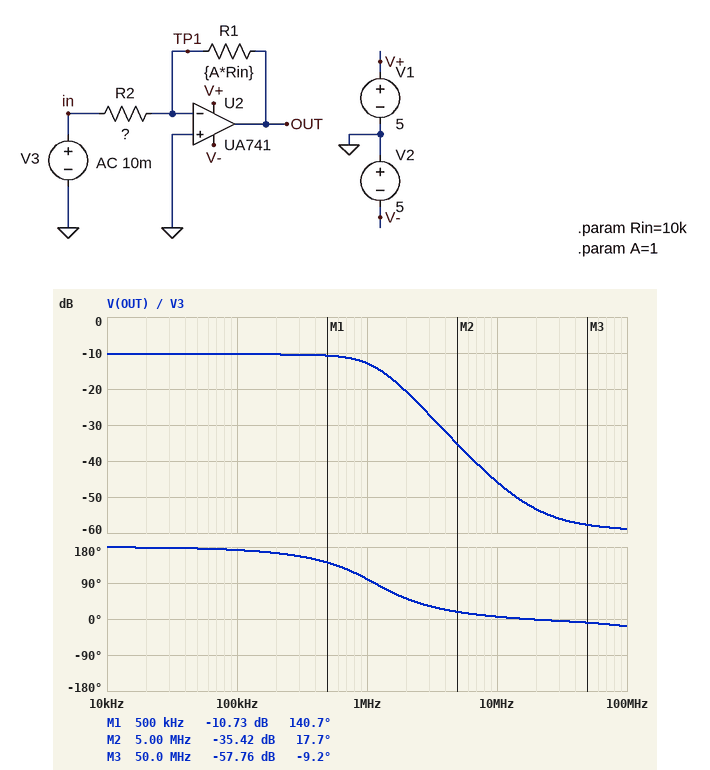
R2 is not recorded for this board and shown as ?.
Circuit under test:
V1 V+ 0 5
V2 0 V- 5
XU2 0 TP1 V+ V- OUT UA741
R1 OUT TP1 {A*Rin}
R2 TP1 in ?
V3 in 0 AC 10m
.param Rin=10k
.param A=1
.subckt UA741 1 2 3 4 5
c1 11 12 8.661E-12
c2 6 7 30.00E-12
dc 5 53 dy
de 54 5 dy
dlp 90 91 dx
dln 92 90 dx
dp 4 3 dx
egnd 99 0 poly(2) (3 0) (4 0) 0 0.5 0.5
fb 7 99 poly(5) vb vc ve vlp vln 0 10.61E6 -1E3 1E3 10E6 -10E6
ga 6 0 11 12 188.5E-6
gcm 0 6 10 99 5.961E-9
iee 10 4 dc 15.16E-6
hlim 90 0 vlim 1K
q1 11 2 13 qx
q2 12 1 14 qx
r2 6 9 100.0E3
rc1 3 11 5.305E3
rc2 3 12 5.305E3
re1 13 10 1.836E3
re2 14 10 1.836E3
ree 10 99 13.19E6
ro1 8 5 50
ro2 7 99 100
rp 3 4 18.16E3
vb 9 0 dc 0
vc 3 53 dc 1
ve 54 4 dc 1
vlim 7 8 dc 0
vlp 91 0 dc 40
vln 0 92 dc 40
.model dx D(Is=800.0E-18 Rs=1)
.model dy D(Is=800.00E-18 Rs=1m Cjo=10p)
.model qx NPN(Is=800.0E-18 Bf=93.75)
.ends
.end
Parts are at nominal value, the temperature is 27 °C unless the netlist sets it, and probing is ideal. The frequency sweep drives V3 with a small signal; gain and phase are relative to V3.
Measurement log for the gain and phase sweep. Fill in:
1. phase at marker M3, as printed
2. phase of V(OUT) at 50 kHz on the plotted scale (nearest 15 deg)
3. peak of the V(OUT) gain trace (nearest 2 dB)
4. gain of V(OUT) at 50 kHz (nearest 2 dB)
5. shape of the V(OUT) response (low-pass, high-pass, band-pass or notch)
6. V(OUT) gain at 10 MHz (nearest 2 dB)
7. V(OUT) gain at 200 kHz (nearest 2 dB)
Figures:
-9.2 deg
180 deg
-10 dB
-10 dB
low-pass
-46 dB
-10 dB
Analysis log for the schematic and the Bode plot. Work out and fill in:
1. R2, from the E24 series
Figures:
33 kΩ
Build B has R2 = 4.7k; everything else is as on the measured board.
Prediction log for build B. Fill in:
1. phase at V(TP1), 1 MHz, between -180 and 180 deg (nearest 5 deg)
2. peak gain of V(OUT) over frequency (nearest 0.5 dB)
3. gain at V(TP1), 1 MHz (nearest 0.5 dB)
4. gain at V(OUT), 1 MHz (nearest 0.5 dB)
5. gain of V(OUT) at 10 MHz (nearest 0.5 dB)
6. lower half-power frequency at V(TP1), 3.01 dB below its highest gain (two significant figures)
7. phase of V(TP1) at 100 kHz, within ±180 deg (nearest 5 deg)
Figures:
15 deg
6.5 dB
-2.5 dB
-3.5 dB
-36.5 dB
320 kHz
75 deg
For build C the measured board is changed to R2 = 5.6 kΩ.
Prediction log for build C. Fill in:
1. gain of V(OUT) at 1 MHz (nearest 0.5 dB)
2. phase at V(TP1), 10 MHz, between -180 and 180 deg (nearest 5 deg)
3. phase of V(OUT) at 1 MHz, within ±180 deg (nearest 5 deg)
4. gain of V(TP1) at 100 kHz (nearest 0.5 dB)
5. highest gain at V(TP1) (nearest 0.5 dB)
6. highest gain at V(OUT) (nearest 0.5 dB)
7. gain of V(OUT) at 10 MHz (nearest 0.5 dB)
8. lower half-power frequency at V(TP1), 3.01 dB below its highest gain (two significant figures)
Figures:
-4.0 dB
0 deg
75 deg
-15.0 dB
-3.0 dB
5.0 dB
-37.0 dB
360 kHz
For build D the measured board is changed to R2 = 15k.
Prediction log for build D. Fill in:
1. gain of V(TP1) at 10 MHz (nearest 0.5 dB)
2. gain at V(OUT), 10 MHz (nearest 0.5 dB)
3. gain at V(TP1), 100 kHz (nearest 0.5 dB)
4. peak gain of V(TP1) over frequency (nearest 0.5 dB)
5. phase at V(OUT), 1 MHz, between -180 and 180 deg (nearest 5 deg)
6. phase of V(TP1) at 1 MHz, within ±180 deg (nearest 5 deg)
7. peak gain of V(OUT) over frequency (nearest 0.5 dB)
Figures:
-8.0 dB
-41.0 dB
-23.5 dB
-6.5 dB
90 deg
30 deg
-3.5 dB
